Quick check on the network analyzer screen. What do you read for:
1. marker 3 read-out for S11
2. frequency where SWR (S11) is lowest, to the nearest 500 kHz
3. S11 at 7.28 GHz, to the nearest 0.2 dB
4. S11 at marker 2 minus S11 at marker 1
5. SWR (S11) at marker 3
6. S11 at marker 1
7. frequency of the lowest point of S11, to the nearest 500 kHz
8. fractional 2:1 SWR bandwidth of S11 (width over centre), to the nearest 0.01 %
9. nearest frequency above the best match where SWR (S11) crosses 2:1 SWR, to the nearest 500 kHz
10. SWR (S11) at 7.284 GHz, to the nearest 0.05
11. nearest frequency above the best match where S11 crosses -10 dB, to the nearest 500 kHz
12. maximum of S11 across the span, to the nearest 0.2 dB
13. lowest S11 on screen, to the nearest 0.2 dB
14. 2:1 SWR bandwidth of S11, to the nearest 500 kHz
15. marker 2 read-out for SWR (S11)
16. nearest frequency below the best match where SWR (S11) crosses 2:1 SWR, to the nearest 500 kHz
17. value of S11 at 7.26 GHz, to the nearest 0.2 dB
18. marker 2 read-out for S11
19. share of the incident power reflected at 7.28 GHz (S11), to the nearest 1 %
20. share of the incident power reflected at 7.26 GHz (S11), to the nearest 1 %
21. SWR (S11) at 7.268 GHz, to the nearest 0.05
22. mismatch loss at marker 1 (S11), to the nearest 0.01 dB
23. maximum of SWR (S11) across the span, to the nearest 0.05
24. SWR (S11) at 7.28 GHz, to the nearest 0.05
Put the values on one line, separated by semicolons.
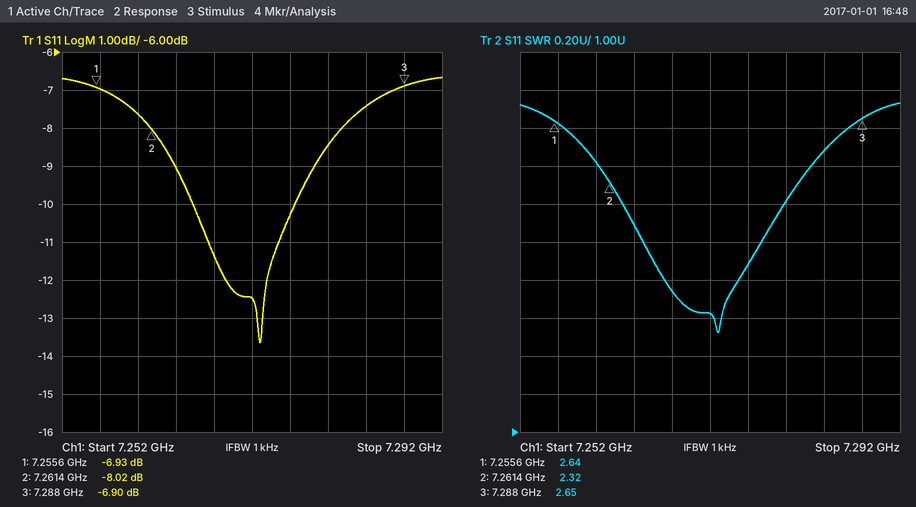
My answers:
-6.90 dB; 7.2730 GHz; -8.4 dB; -1.09 dB; 2.65; -6.93 dB; 7.2730 GHz; 0.17 %; 7.2775 GHz; 2.50; 7.2765 GHz; -6.6 dB; -13.6 dB; 12.5 MHz; 2.32; 7.2650 GHz; -7.6 dB; -8.02 dB; 14 %; 17 %; 1.75; 0.98 dB; 2.75; 2.20
